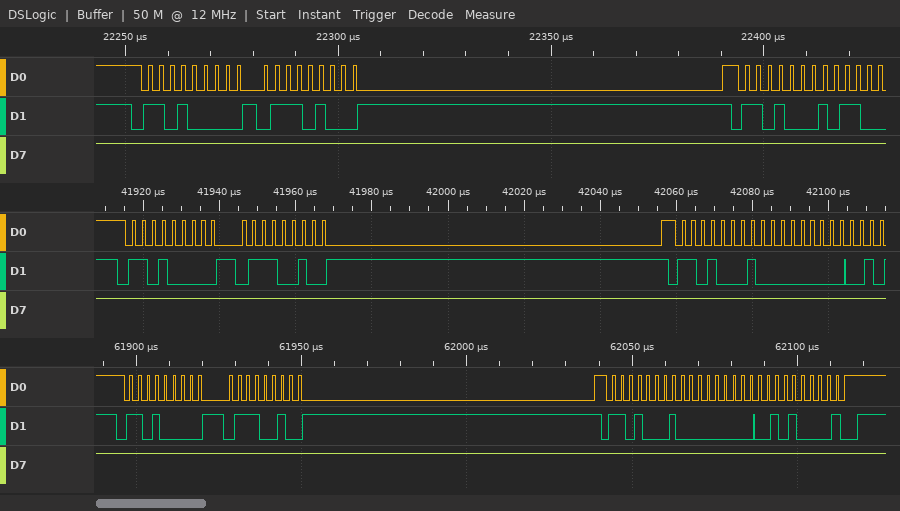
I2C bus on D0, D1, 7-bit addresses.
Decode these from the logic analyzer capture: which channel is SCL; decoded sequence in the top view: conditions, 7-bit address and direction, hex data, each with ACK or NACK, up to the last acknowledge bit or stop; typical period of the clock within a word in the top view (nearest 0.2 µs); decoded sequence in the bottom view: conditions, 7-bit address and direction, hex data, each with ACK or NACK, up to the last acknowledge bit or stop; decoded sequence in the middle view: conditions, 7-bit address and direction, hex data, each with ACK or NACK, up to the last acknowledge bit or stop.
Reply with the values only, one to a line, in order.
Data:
D0
start, address 68 write ACK, 74 ACK, repeated start, address 68 read ACK
2.6 µs
start, address 68 write ACK, 72 ACK, repeated start, address 68 read ACK, 00 ACK, 50 NACK, stop
start, address 68 write ACK, 72 ACK, repeated start, address 68 read ACK, 00 ACK
